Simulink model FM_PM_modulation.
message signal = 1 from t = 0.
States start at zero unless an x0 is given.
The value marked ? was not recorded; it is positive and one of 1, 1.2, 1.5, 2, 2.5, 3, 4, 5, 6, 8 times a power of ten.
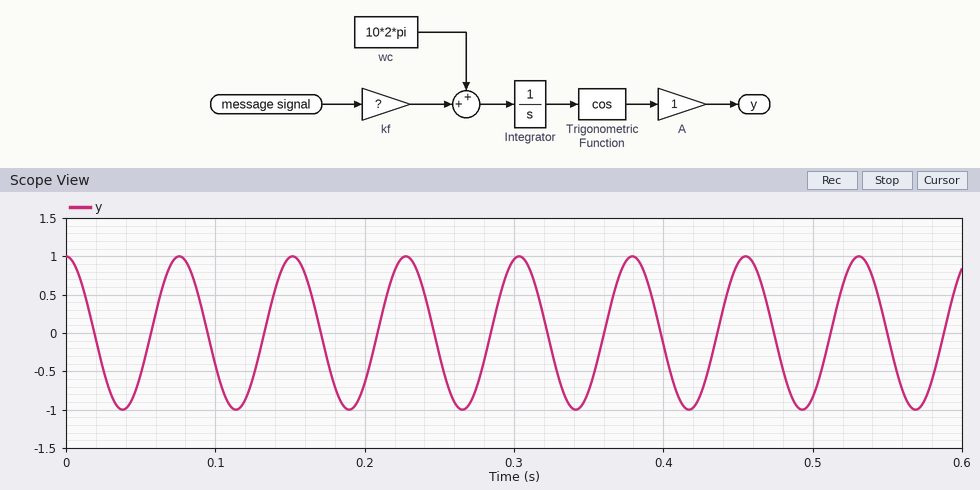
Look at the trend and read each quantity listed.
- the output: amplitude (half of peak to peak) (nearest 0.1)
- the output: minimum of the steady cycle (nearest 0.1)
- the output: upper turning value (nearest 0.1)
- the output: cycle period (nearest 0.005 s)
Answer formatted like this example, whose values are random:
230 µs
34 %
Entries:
1.0
-1.0
1.0
0.075 s
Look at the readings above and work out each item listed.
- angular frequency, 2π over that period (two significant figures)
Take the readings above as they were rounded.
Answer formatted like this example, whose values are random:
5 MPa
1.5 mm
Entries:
84 rad/s
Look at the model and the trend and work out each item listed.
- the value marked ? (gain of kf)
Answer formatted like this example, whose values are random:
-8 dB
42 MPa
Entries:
20
